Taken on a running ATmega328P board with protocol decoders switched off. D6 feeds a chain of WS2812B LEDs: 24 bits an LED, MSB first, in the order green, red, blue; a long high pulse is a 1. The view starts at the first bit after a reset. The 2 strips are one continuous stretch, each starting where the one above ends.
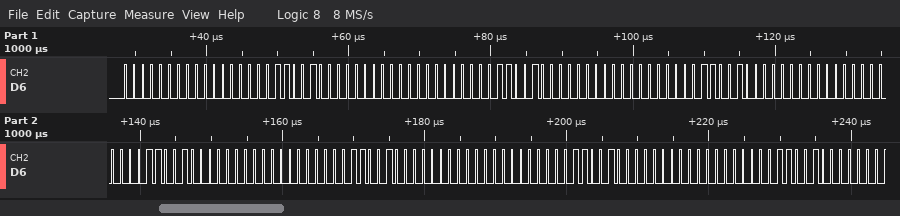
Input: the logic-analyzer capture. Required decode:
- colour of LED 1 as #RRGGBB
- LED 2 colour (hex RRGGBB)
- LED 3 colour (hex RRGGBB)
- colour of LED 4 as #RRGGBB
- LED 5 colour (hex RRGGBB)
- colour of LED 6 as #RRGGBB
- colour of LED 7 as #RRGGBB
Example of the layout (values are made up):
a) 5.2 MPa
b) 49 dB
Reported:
a) #000064
b) #000032
c) #000064
d) #000032
e) #000064
f) #000032
g) #000064
